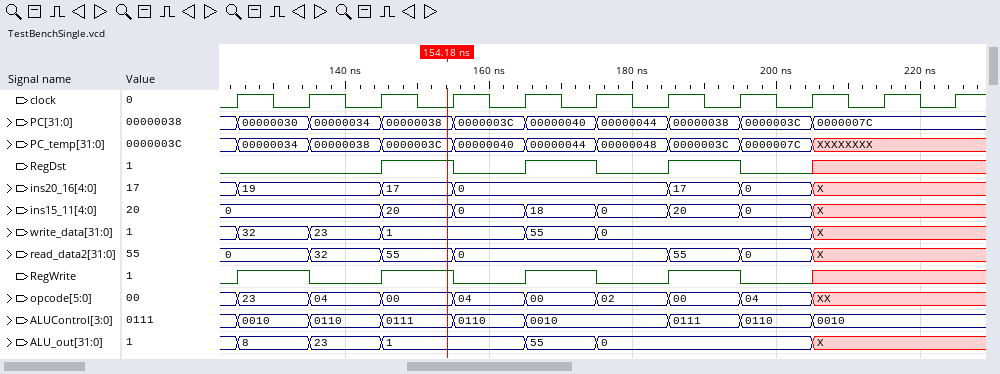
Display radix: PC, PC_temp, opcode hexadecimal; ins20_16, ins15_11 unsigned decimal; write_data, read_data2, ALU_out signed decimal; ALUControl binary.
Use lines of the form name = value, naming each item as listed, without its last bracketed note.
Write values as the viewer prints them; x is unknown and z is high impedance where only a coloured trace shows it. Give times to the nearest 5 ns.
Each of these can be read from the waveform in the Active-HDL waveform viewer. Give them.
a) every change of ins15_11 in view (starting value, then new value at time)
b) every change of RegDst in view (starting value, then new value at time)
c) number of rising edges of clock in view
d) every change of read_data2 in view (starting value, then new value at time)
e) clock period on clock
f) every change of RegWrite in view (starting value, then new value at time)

every change of ins15_11 in view = 0, 20 at 145 ns, 0 at 155 ns, 18 at 165 ns, 0 at 175 ns, 20 at 185 ns, 0 at 195 ns, X at 205 ns
every change of RegDst in view = 0, 1 at 145 ns, 0 at 155 ns, 1 at 165 ns, 0 at 175 ns, 1 at 185 ns, 0 at 195 ns, x at 205 ns
number of rising edges of clock in view = 11
every change of read_data2 in view = 0, 32 at 135 ns, 55 at 145 ns, 0 at 155 ns, 55 at 185 ns, 0 at 195 ns, X at 205 ns
clock period on clock = 10 ns
every change of RegWrite in view = 0, 1 at 125 ns, 0 at 135 ns, 1 at 145 ns, 0 at 155 ns, 1 at 165 ns, 0 at 175 ns, 1 at 185 ns, 0 at 195 ns, x at 205 ns
